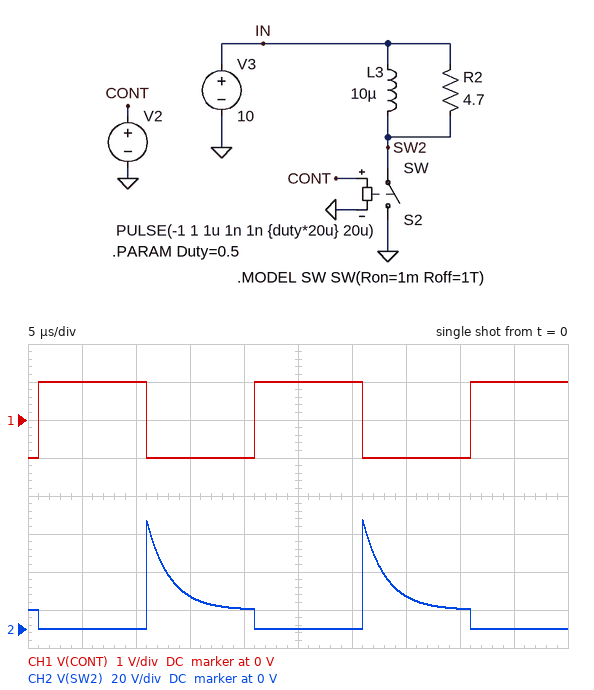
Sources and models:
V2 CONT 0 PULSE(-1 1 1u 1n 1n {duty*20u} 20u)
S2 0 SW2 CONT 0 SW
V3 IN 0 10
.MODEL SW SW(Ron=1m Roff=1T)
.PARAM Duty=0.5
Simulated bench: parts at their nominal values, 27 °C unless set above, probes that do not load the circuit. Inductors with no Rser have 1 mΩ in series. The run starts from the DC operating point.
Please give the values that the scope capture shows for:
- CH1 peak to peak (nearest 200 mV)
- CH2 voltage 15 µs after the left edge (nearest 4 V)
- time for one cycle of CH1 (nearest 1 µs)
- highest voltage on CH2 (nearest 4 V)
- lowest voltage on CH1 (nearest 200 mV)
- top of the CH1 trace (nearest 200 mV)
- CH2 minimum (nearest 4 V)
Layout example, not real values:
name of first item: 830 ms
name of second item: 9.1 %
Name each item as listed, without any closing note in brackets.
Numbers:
CH1 peak to peak: 2.0 V
CH2 voltage 15 µs after the left edge: 16 V
time for one cycle of CH1: 20 µs
highest voltage on CH2: 56 V
lowest voltage on CH1: -1.0 V
top of the CH1 trace: 1.0 V
CH2 minimum: 0 V
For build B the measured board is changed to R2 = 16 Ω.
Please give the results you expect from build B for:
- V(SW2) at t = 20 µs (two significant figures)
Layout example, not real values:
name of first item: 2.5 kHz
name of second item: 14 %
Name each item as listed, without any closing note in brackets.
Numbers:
V(SW2) at t = 20 µs: 10 V
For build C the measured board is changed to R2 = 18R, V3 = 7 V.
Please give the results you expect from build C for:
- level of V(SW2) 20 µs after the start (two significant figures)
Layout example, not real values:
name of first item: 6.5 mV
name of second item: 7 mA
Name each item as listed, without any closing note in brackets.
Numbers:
level of V(SW2) 20 µs after the start: 7.0 V
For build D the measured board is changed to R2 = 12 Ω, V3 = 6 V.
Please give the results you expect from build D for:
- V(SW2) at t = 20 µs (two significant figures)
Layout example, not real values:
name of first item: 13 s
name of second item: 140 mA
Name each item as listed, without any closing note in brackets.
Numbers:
V(SW2) at t = 20 µs: 6.0 V
